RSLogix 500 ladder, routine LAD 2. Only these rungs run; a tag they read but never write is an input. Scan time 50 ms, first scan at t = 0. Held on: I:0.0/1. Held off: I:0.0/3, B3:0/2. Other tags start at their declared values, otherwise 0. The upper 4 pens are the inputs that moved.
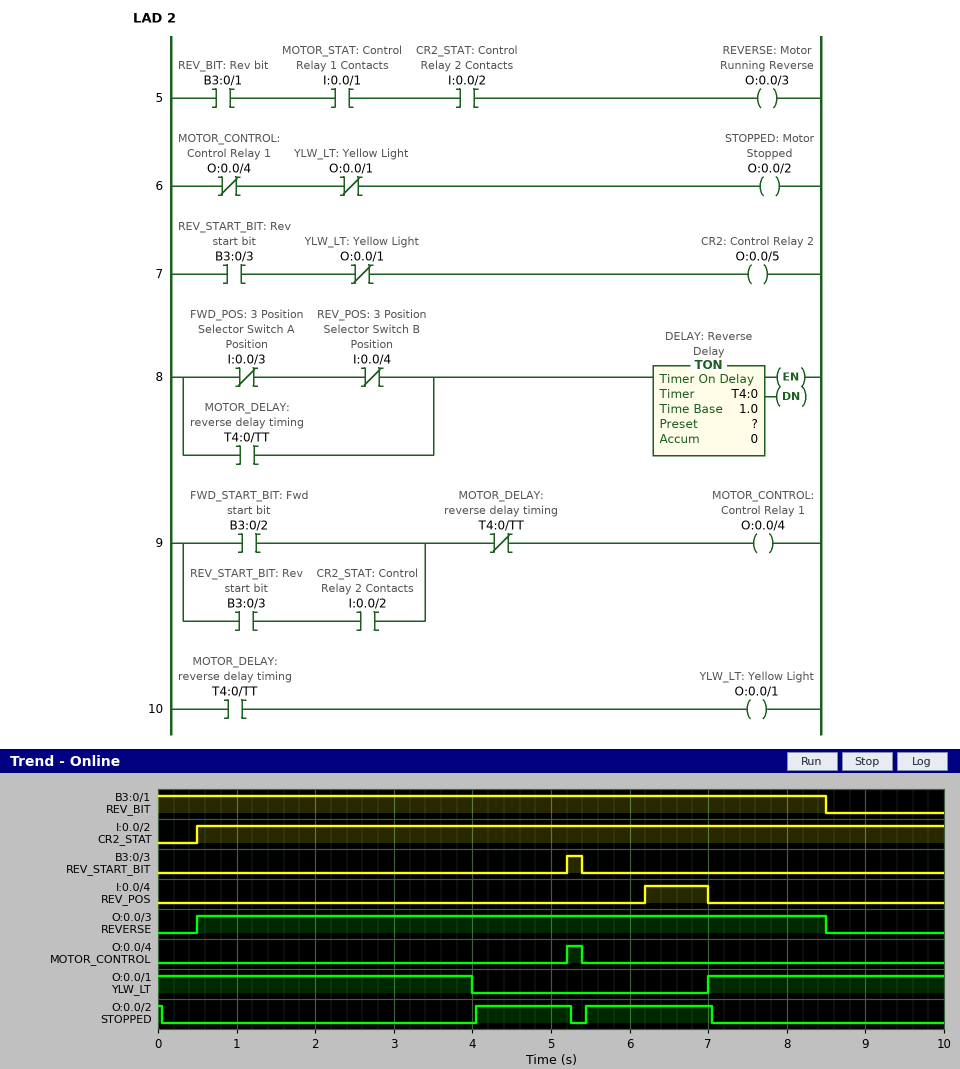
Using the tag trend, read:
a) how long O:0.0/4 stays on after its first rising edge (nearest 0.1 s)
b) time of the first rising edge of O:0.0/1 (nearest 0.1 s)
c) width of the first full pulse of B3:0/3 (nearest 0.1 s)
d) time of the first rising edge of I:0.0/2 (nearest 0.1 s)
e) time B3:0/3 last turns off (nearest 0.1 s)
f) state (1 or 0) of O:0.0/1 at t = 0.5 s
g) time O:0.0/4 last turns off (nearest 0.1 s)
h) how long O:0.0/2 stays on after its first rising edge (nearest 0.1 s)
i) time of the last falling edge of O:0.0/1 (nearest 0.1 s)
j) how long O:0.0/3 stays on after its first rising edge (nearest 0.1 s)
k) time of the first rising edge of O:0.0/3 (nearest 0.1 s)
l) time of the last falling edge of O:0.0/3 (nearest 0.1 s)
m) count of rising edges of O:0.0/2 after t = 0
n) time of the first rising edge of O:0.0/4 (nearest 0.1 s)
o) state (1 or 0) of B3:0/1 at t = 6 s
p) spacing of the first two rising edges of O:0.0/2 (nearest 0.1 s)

0.2 s
7.0 s
0.2 s
0.5 s
5.4 s
1
5.4 s
1.2 s
4.0 s
8.0 s
0.5 s
8.5 s
2
5.2 s
1
1.4 s
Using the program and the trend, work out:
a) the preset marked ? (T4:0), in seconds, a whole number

4 s
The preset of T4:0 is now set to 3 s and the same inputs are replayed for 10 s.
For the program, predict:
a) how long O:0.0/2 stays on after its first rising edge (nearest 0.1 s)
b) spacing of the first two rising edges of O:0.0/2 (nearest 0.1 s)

2.2 s
2.4 s
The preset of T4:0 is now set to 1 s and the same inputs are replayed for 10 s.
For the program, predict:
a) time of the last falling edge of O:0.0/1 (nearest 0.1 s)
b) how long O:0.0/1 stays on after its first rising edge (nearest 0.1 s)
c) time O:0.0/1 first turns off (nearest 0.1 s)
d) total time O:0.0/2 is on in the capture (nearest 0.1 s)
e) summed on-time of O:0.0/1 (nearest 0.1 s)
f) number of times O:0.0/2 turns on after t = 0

8.0 s
1.0 s
1.0 s
7.8 s
2.0 s
3
